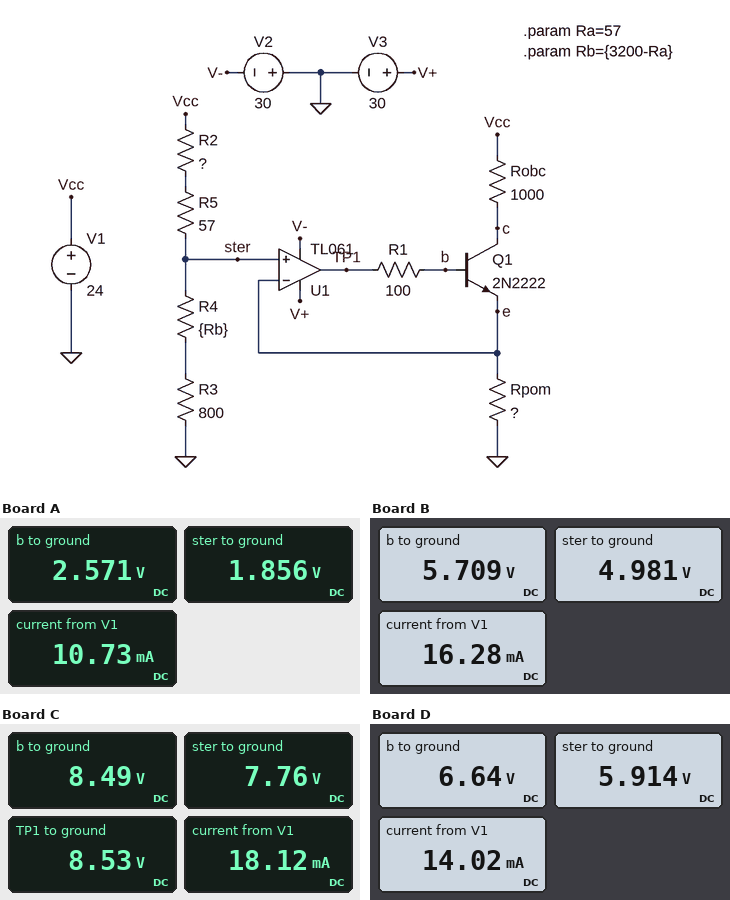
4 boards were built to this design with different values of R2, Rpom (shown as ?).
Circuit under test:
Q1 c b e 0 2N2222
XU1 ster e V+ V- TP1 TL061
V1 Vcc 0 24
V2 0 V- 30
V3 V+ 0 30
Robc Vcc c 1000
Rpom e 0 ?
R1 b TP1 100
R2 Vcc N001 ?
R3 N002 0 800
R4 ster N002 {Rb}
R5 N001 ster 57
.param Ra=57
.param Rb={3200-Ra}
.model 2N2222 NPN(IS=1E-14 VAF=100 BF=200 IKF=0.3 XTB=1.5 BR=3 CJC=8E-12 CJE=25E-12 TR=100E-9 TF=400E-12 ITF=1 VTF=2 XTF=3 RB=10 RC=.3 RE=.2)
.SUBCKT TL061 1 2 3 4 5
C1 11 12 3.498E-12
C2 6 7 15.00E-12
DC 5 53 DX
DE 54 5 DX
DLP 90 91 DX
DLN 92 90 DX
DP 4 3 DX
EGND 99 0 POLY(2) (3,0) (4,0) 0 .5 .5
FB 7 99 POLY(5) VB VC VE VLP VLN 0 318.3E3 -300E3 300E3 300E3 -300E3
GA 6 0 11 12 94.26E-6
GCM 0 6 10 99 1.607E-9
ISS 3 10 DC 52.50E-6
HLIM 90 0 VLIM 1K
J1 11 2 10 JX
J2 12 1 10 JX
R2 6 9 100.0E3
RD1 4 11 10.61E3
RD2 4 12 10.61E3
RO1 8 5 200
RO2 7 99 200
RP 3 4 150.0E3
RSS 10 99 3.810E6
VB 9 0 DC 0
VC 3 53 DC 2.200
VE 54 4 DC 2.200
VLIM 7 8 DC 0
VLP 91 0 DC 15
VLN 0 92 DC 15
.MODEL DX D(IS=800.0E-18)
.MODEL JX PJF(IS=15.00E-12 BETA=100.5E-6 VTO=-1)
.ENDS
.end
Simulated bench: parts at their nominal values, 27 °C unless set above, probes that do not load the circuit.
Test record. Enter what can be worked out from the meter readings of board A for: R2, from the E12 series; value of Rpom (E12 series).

47 kΩ
180 Ω
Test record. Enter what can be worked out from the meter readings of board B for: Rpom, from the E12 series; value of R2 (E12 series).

330 Ω
15 kΩ
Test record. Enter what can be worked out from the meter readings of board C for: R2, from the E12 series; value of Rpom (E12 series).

8.2 kΩ
470 Ω
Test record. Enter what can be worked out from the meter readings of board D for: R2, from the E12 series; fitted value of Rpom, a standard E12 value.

12 kΩ
470 Ω
